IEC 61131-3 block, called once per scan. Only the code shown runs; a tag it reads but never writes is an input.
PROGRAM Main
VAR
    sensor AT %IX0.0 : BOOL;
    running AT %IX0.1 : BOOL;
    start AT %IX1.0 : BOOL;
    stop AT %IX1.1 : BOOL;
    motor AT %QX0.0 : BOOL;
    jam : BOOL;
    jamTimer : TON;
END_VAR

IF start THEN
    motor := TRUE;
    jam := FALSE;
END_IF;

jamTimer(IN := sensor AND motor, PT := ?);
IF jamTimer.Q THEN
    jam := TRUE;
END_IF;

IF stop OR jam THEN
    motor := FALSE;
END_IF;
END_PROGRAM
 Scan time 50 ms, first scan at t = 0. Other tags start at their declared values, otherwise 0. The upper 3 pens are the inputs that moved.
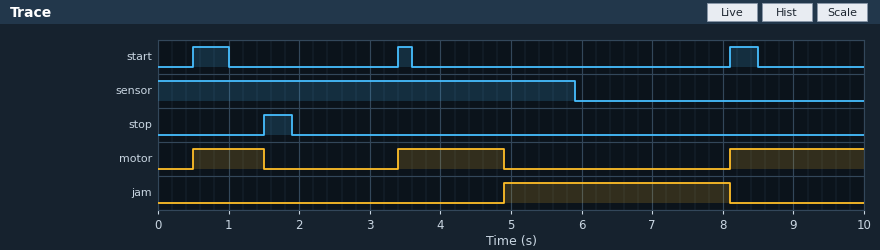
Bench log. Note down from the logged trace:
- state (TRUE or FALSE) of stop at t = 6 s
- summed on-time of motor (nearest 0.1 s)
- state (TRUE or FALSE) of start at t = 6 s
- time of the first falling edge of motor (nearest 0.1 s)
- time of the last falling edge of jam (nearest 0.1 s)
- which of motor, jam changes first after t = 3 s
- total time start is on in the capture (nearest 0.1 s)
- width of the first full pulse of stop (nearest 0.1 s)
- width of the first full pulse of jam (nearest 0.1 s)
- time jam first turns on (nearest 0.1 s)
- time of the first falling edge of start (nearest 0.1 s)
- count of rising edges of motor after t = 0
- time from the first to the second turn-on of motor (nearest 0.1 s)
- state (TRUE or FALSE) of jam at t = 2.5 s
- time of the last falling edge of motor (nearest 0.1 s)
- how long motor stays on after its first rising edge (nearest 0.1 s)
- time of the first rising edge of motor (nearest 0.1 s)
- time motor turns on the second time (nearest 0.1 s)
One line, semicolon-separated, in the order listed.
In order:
FALSE; 4.4 s; FALSE; 1.5 s; 8.1 s; motor; 1.1 s; 0.4 s; 3.2 s; 4.9 s; 1.0 s; 3; 2.9 s; FALSE; 4.9 s; 1.0 s; 0.5 s; 3.4 s
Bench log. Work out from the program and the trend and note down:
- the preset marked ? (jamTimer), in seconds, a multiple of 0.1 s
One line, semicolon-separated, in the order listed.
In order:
1.5 s
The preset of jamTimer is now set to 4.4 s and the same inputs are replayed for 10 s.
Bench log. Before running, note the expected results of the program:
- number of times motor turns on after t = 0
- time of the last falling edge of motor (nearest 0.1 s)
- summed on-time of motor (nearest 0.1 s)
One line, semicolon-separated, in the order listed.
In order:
2; 1.5 s; 7.6 s
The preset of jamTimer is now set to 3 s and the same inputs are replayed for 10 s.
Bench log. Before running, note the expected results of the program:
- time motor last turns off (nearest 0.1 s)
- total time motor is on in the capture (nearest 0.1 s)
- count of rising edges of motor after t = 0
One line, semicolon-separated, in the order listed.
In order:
1.5 s; 7.6 s; 2
